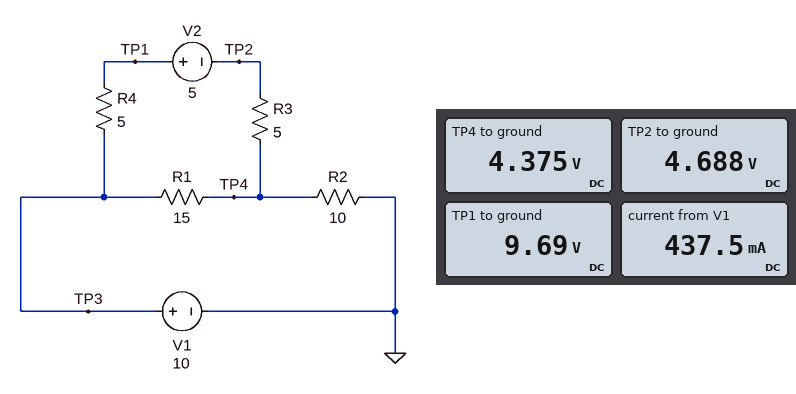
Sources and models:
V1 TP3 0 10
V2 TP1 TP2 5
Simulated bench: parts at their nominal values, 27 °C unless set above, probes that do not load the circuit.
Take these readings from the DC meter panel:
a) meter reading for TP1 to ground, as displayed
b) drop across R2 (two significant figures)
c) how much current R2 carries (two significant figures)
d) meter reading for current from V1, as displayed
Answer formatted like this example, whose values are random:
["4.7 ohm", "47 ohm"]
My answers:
["9.69 V", "4.4 V", "440 mA", "437.5 mA"]
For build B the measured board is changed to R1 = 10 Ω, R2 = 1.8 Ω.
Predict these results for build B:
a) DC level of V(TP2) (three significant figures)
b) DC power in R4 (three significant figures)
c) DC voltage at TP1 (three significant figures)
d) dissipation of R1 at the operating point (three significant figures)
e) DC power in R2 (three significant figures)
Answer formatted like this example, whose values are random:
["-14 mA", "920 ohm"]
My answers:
["3.49 V", "454 mW", "8.49 V", "6.42 W", "2.19 W"]
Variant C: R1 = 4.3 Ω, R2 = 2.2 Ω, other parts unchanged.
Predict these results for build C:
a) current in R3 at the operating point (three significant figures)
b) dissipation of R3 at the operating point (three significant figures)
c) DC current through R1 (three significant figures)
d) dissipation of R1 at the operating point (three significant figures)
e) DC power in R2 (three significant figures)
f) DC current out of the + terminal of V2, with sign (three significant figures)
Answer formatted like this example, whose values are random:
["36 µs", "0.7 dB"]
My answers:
["141 mA", "99.4 mW", "1.49 A", "9.56 W", "5.86 W", "-141 mA"]
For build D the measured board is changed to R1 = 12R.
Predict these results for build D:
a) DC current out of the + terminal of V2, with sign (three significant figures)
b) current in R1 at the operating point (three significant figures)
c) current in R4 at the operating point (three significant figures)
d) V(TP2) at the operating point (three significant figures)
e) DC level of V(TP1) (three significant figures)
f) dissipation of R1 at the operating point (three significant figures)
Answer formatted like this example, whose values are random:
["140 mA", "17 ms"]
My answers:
["-29.4 mA", "441 mA", "29.4 mA", "4.85 V", "9.85 V", "2.34 W"]
